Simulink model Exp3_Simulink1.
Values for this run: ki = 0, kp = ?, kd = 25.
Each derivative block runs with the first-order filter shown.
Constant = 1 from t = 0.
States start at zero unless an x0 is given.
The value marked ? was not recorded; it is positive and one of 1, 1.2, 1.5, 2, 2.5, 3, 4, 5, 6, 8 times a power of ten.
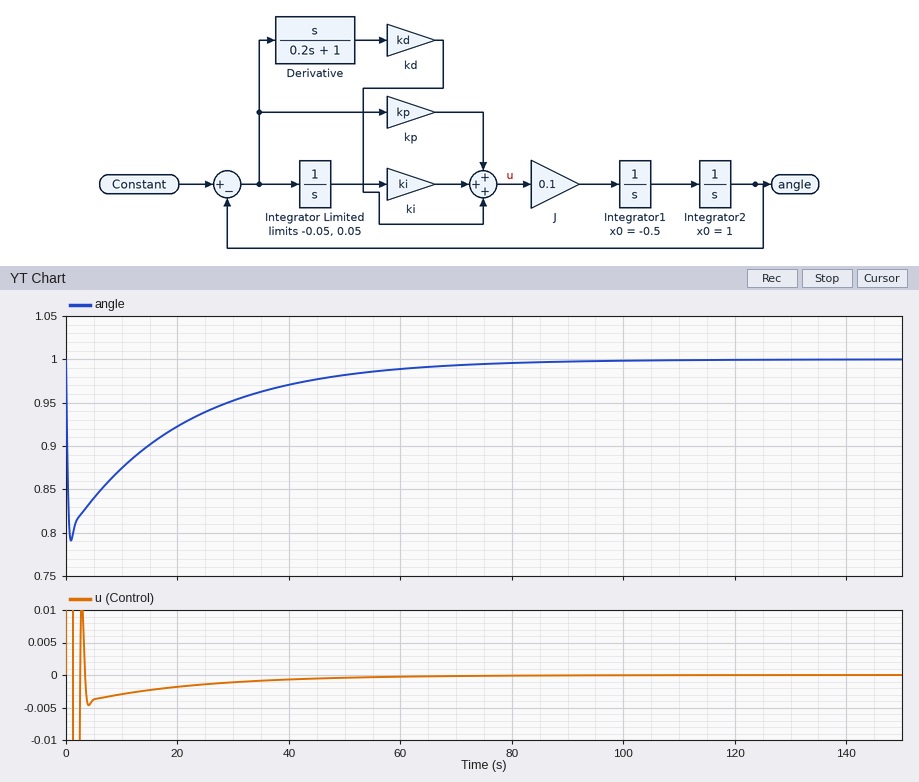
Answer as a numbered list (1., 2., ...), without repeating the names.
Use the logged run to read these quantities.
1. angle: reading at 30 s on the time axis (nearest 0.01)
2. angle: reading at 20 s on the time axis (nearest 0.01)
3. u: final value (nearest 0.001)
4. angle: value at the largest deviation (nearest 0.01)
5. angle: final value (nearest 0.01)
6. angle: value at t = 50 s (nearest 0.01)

1. 0.95
2. 0.92
3. 0.000
4. 0.79
5. 1.00
6. 0.98
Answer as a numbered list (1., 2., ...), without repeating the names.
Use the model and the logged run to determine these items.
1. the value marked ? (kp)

1. 1.2
